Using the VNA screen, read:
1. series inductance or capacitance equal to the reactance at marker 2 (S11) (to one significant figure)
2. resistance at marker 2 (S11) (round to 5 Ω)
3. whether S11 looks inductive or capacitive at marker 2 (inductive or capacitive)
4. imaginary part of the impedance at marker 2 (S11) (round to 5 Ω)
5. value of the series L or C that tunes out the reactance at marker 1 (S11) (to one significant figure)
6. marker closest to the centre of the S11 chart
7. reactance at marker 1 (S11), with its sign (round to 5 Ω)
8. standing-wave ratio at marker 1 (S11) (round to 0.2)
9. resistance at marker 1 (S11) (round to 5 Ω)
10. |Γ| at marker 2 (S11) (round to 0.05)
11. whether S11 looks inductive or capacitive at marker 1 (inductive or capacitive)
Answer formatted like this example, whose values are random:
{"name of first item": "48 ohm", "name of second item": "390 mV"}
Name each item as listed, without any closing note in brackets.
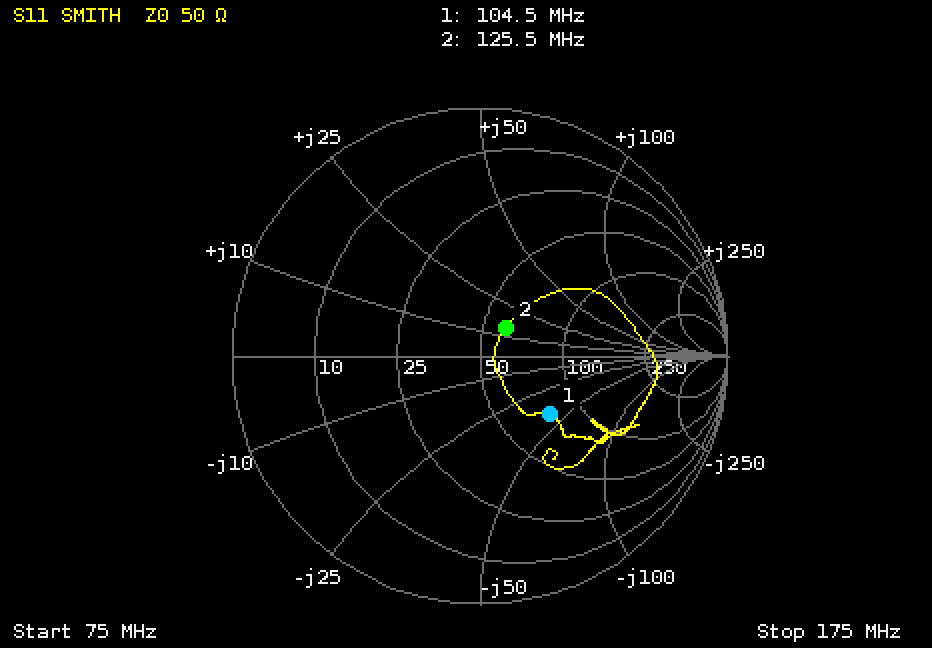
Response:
{"series inductance or capacitance equal to the reactance at marker 2 (S11)": "20 nH", "resistance at marker 2 (S11)": "60 Ω", "whether S11 looks inductive or capacitive at marker 2": "inductive", "imaginary part of the impedance at marker 2 (S11)": "+15 Ω", "value of the series L or C that tunes out the reactance at marker 1 (S11)": "60 nH", "marker closest to the centre of the S11 chart": "marker 2", "reactance at marker 1 (S11), with its sign": "-40 Ω", "standing-wave ratio at marker 1 (S11)": "2.2", "resistance at marker 1 (S11)": "75 Ω", "|Γ| at marker 2 (S11)": "0.15", "whether S11 looks inductive or capacitive at marker 1": "capacitive"}
